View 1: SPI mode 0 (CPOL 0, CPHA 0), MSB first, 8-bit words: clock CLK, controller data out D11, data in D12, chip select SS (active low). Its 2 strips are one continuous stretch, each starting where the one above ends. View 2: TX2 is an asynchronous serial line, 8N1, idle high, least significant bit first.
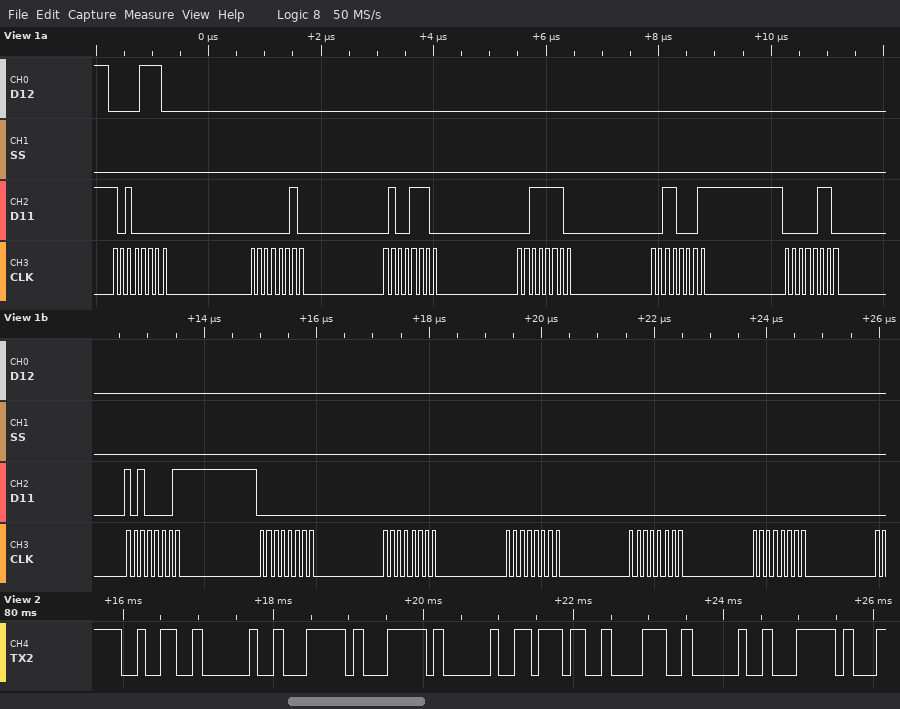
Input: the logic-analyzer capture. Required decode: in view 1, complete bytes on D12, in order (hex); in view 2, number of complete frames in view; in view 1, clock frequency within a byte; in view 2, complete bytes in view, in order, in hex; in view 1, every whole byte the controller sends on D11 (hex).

0E 00 00 00 00 00 00 00 00 00 00 00
9
8 MHz
32 20 7C 7C 20 37 38 20 7C
A0 02 4E 3E 31 06 A1 00 00 00 00 00
